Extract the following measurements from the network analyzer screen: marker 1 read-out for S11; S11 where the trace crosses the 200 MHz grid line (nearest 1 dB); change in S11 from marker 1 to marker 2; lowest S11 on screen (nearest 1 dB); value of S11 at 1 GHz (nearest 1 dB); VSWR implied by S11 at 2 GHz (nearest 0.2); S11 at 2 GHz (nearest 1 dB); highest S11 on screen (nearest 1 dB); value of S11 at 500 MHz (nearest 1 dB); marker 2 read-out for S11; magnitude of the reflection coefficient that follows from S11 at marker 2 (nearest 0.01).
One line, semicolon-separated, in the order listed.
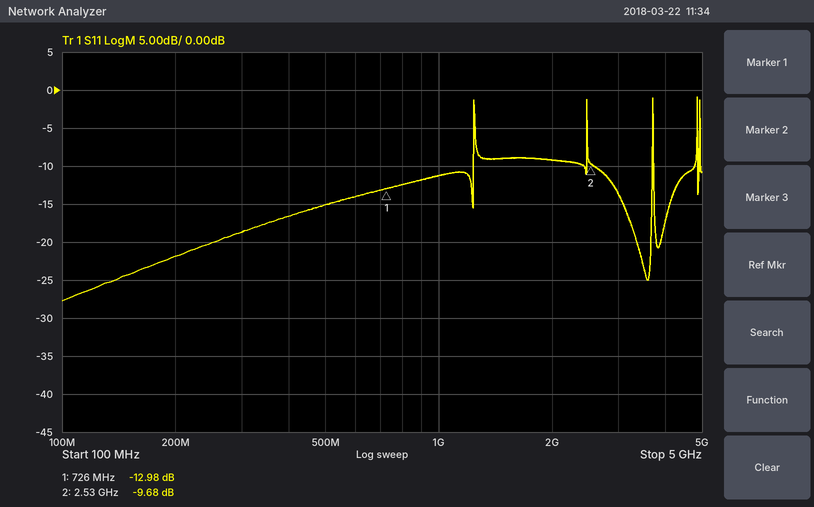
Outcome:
-12.98 dB; -22 dB; 3.30 dB; -28 dB; -11 dB; 2.0; -9 dB; -1 dB; -15 dB; -9.68 dB; 0.33
